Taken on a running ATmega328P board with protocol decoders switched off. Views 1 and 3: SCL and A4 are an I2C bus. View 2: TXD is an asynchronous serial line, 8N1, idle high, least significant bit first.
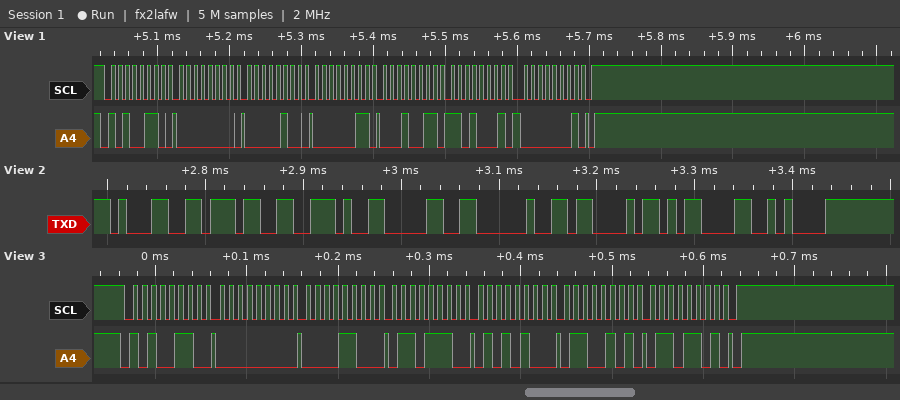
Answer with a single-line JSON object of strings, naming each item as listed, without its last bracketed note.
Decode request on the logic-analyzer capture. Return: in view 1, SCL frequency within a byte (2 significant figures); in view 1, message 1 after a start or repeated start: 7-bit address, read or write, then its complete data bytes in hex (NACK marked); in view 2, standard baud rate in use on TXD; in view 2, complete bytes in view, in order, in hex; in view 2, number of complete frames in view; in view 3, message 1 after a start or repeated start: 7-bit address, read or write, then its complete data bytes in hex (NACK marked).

{"in view 1, SCL frequency within a byte": "100 kHz", "in view 1, message 1 after a start or repeated start: 7-bit address, read or write, then its complete data bytes in hex": "0x53 write: 00 04 03 13 D1 01", "in view 2, standard baud rate in use on TXD": "115200 baud", "in view 2, complete bytes in view, in order, in hex": "31 37 2E 30 20 43 0D 0A", "in view 2, number of complete frames in view": "8", "in view 3, message 1 after a start or repeated start: 7-bit address, read or write, then its complete data bytes in hex": "0x53 write: 00 0C 6E 54 65 6D"}
